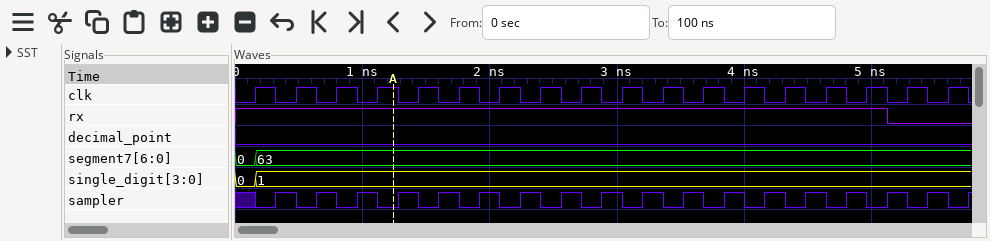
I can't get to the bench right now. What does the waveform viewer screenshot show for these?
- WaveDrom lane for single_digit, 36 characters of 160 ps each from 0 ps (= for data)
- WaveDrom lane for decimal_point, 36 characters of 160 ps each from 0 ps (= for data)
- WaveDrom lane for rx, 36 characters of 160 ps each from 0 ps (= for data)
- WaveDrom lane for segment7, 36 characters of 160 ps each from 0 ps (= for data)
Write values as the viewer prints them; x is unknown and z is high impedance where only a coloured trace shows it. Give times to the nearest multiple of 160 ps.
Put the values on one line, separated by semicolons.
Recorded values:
{name: 'single_digit', wave: '==..................................', data: '0 1'}; {name: 'decimal_point', wave: '0...................................'}; {name: 'rx', wave: '1...............................0...'}; {name: 'segment7', wave: '==..................................', data: '0 63'}
